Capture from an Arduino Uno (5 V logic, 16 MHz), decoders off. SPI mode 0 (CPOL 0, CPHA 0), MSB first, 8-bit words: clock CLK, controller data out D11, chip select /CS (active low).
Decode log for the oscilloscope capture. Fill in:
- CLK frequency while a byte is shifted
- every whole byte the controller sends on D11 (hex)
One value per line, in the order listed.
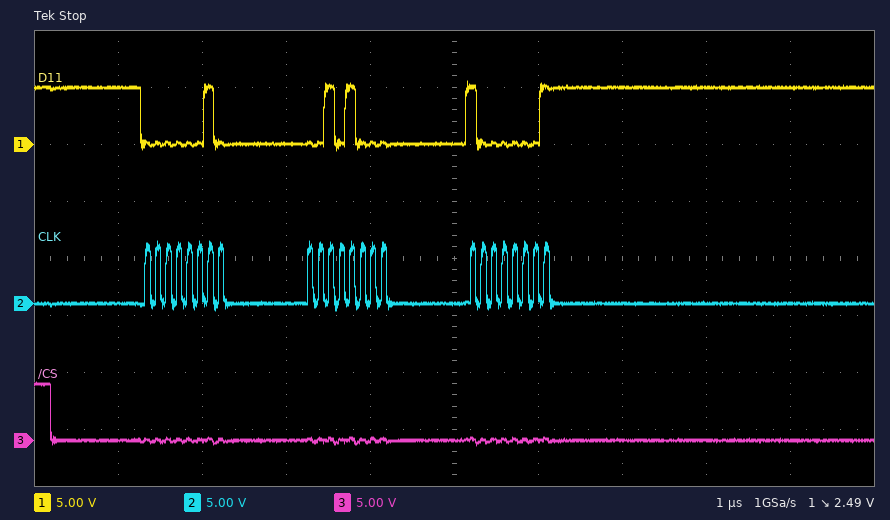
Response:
8 MHz
0x02 0x28 0x81
